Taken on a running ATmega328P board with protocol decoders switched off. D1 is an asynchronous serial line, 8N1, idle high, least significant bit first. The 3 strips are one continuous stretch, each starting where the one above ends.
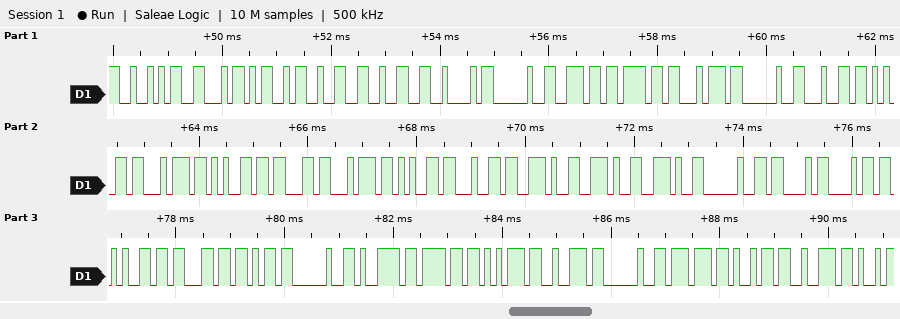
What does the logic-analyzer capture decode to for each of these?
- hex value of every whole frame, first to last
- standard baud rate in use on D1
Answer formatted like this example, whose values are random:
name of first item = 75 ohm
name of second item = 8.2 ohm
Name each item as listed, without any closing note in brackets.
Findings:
hex value of every whole frame, first to last = 52 46 4D 32 32 42 20 6E 6F 74 20 64 65 74 65 63 74 65 64 2E 2E 2E 20 43 68 65 63 6B 20 79 6F 75 72 20 77 69 72
standard baud rate in use on D1 = 9600 baud
